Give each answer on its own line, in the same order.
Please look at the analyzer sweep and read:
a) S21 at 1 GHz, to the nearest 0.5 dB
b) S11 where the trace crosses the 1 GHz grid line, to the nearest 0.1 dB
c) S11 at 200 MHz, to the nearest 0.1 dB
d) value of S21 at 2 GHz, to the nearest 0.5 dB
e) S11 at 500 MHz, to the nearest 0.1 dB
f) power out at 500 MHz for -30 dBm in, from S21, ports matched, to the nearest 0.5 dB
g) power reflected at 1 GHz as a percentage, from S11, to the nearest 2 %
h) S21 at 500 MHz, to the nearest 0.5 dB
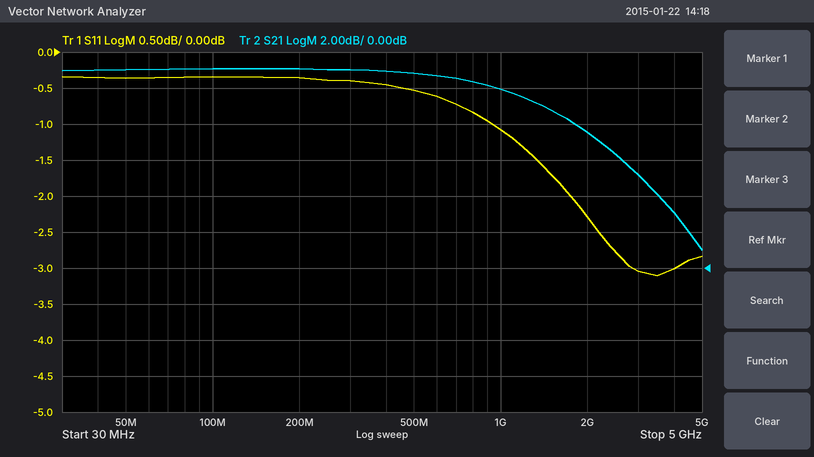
10.0 dB
-1.1 dB
-0.4 dB
7.5 dB
-0.5 dB
-19.0 dBm
78 %
11.0 dB
